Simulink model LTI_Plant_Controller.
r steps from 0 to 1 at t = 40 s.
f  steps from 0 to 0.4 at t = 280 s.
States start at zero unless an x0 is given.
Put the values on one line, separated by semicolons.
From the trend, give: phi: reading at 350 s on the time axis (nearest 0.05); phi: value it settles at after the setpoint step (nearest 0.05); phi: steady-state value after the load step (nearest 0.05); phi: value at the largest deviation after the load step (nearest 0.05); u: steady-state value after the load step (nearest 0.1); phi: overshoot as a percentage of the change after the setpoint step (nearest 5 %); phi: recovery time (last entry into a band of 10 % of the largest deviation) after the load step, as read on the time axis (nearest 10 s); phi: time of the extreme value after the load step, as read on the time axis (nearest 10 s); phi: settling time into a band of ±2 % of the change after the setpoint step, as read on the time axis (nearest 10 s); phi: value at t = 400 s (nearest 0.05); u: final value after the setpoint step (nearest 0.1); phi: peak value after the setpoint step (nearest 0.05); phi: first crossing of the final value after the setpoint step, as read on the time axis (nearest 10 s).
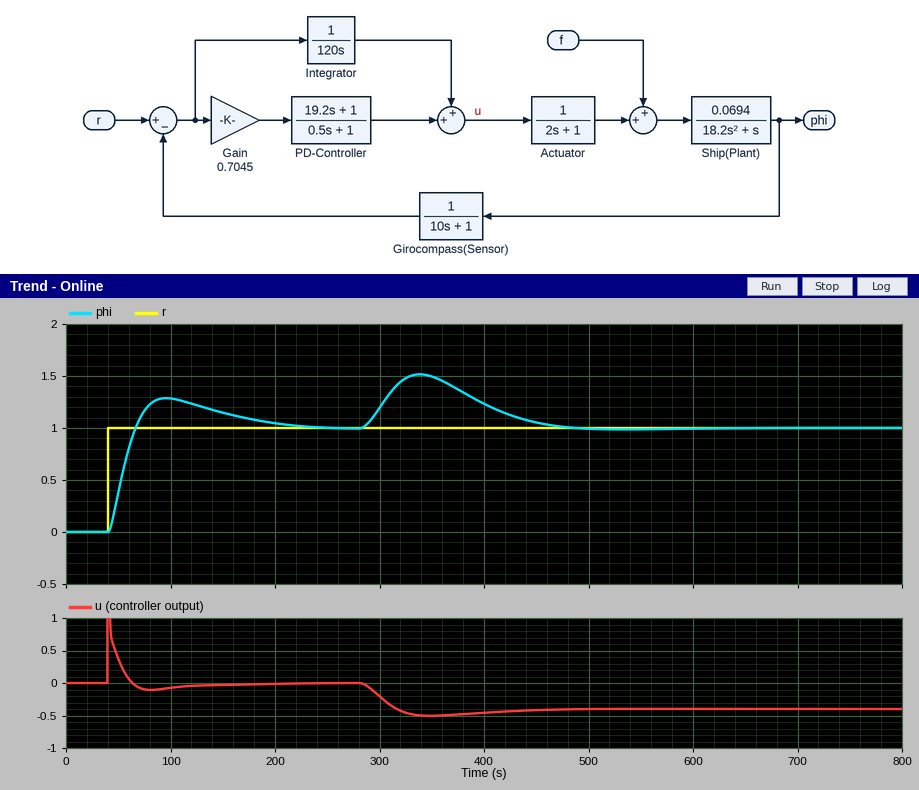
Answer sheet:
1.50; 1.00; 1.00; 1.50; -0.4; 30 %; 450 s; 340 s; 220 s; 1.25; 0.0; 1.30; 70 s
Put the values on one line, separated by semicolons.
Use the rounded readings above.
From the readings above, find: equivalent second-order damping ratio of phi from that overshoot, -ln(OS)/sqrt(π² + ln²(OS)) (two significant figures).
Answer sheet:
0.36
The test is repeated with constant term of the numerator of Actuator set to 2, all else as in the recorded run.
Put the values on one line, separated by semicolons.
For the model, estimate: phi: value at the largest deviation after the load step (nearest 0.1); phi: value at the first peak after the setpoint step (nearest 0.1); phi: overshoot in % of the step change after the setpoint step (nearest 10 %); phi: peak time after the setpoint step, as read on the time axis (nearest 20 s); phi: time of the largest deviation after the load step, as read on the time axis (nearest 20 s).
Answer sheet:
1.3; 1.5; 50 %; 60 s; 320 s
